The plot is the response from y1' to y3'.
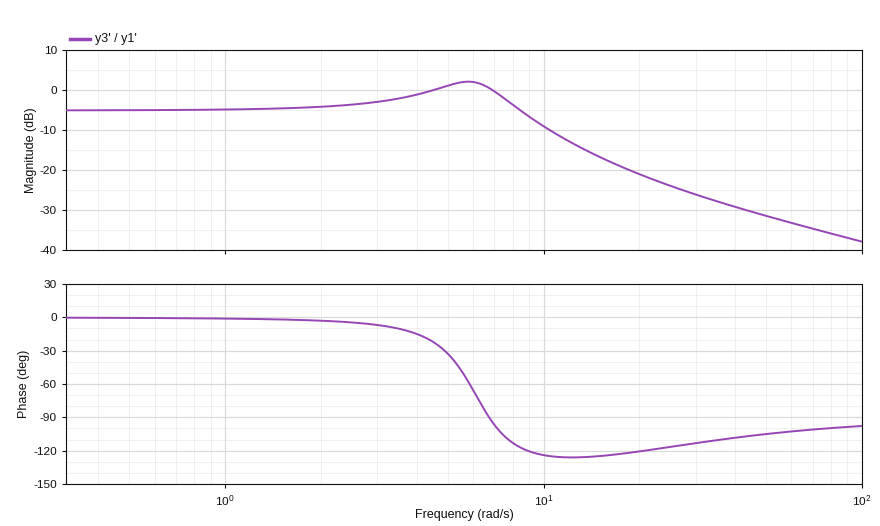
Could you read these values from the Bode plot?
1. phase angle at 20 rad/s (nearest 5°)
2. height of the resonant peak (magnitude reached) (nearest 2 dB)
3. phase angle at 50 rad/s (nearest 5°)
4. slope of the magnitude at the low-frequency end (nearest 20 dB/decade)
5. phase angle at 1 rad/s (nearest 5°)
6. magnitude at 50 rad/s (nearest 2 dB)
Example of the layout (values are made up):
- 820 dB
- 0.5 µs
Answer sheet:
- -120°
- 2 dB
- -105°
- 0 dB/decade
- 0°
- -32 dB
